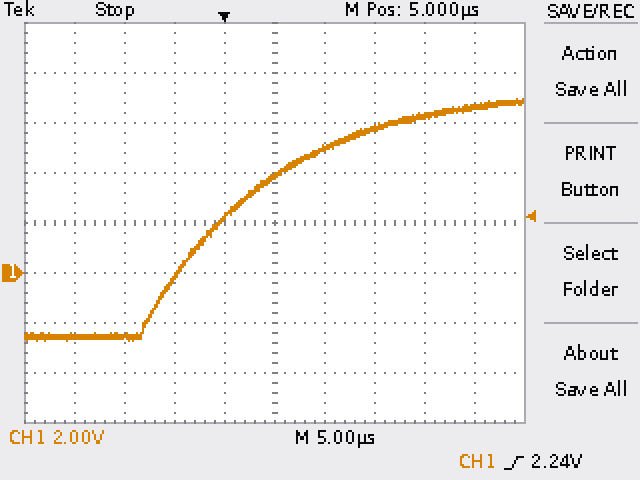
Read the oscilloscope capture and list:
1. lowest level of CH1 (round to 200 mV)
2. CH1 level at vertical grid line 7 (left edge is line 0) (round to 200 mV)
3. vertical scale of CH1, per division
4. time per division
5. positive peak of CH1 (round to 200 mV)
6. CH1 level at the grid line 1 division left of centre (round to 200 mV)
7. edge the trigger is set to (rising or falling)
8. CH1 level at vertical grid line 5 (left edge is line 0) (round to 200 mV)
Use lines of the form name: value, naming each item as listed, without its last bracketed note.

lowest level of CH1: -2.8 V
CH1 level at vertical grid line 7 (left edge is line 0): 5.8 V
vertical scale of CH1, per division: 2 V
time per division: 5 µs
positive peak of CH1: 7.0 V
CH1 level at the grid line 1 division left of centre: 2.2 V
edge the trigger is set to: rising
CH1 level at vertical grid line 5 (left edge is line 0): 3.8 V
